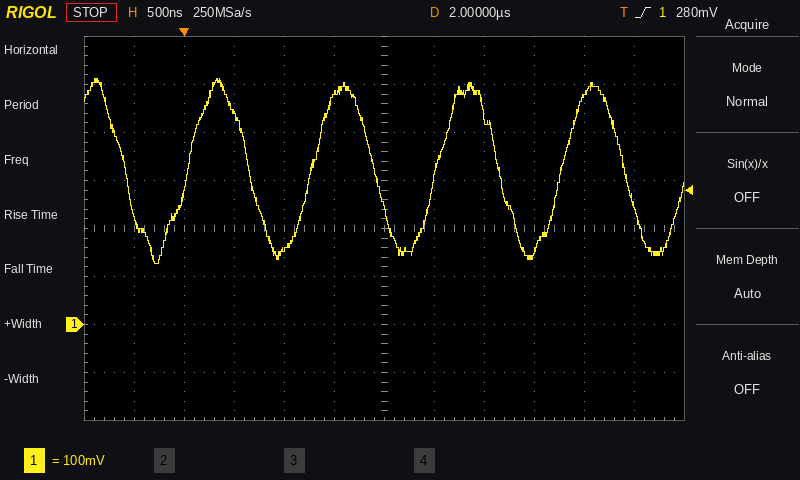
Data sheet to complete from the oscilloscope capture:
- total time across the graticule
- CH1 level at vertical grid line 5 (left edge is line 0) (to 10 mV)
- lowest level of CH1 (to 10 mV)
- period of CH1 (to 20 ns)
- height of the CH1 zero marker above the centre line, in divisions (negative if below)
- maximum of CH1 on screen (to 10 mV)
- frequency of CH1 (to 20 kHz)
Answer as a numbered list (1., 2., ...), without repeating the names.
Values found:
1. 6 µs
2. 480 mV
3. 130 mV
4. 1.24 µs
5. -2.0 div
6. 510 mV
7. 800 kHz
